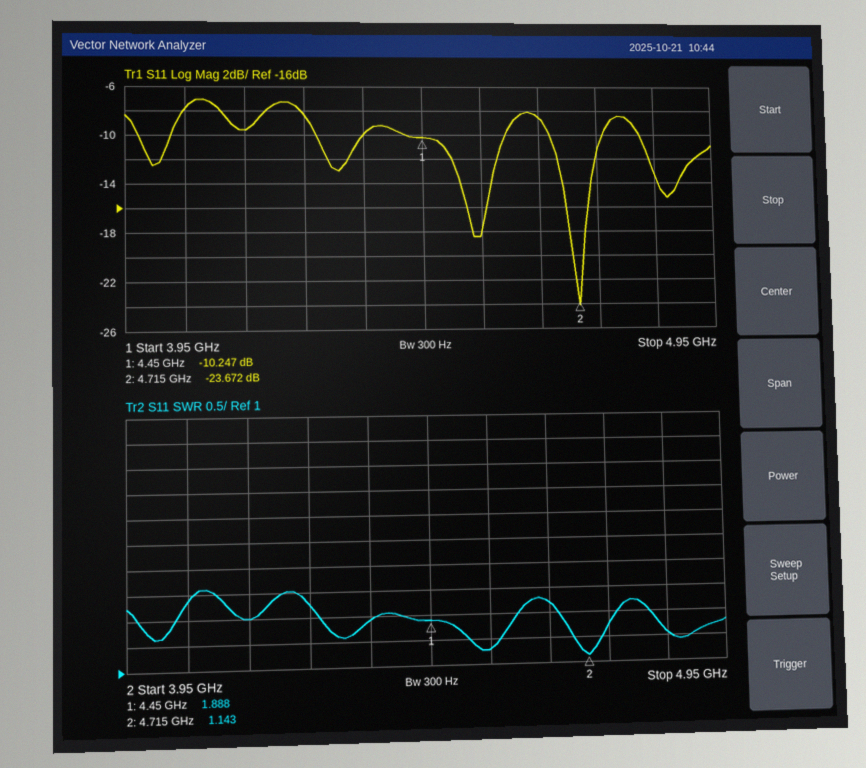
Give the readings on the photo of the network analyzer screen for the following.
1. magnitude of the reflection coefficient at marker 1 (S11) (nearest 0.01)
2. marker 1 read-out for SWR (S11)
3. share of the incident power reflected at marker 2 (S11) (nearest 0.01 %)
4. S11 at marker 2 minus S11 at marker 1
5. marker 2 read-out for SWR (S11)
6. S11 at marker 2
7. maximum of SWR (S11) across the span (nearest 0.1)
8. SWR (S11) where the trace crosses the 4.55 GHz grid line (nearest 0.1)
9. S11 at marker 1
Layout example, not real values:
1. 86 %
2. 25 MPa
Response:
1. 0.31
2. 1.888
3. 0.43 %
4. -13.425 dB
5. 1.143
6. -23.672 dB
7. 2.6
8. 1.3
9. -10.247 dB
